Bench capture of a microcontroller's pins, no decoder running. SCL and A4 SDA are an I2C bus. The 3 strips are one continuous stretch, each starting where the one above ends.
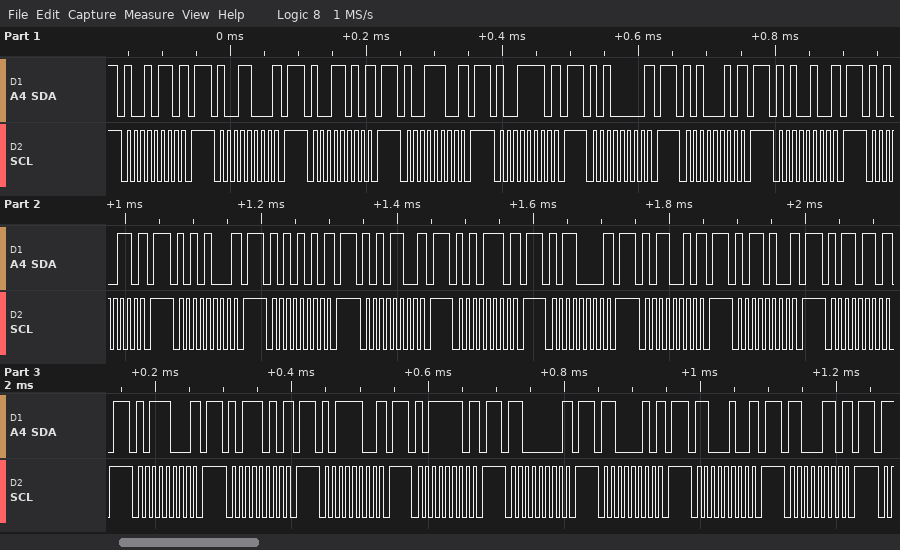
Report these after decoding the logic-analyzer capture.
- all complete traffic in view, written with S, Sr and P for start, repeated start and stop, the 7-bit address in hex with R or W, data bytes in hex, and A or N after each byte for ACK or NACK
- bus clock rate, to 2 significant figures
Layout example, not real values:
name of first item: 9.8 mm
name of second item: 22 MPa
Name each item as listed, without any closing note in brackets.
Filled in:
all complete traffic in view, written with S, Sr and P for start, repeated start and stop, the 7-bit address in hex with R or W, data bytes in hex, and A or N after each byte for ACK or NACK: S 4BW N P S 4CW N P S 4DW N P S 4EW N P S 4FW N P S 50W N P S 51W N P S 52W N P S 53W N P S 54W N P S 55W N P S 56W N P S 57W N P S 58W N P S 59W N P S 5AW N P S 5BW N P S 5CW N P S 5DW N P S 5EW N P S 5FW N P S 60W N P S 61W N P S 62W N P S 63W N P
bus clock rate, to 2 significant figures: 100 kHz
